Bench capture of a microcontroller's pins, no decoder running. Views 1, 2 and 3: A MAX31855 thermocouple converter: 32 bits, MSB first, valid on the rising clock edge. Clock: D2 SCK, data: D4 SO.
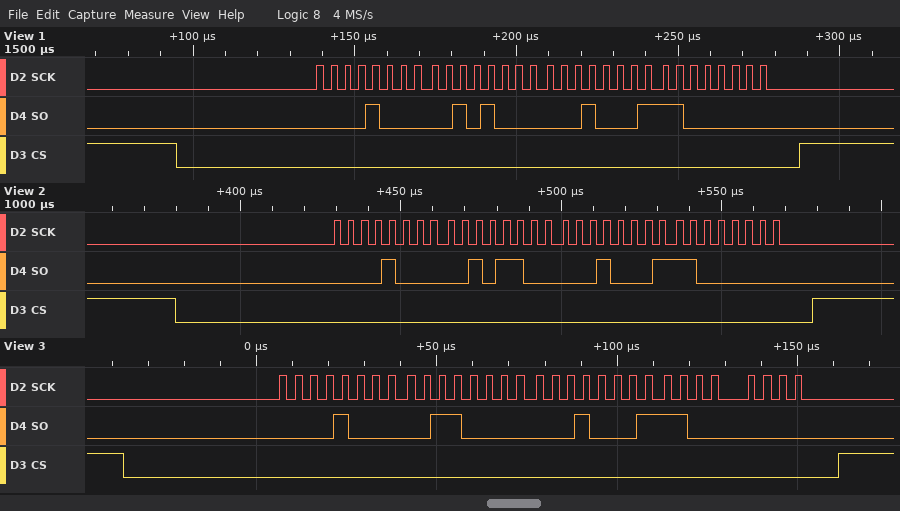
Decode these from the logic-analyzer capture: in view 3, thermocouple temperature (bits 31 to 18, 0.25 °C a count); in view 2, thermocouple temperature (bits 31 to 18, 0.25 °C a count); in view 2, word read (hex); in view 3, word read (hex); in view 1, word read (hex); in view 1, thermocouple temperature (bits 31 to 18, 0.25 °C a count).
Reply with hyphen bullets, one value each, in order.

- 131.00 °C
- 130.75 °C
- 0x082C11C0
- 0x083011C0
- 0x082811C0
- 130.50 °C
